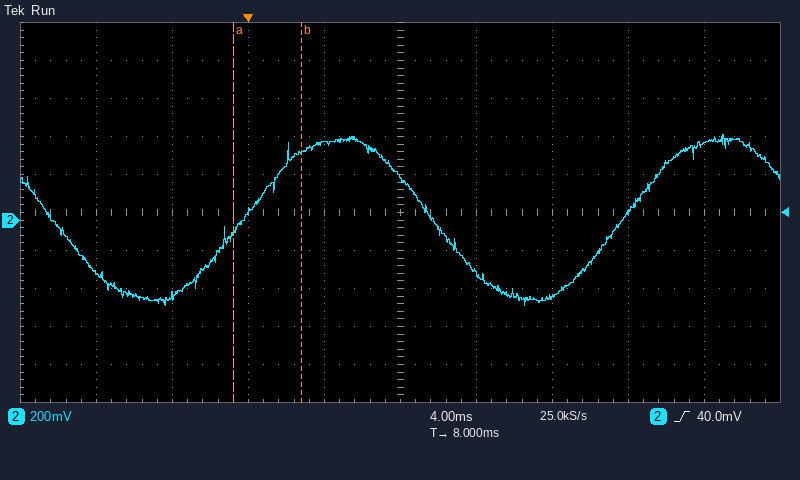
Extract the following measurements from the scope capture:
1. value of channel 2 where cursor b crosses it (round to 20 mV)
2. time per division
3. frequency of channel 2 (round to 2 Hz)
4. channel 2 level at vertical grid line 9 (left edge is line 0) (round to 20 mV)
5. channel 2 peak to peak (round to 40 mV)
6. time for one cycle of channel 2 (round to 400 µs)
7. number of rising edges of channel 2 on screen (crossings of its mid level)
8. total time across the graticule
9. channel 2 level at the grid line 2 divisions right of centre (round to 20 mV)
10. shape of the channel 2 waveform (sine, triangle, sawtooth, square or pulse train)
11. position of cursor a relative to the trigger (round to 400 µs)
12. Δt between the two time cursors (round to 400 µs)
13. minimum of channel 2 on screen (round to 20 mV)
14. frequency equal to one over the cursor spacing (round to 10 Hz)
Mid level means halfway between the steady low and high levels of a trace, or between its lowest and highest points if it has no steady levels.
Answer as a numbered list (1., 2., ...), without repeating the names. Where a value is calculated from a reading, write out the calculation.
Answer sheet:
1. 360 mV
2. 4 ms
3. 1 / 20.0 ms ≈ 50 Hz
4. 400 mV
5. 880 mV
6. 20.0 ms
7. 2
8. 40 ms
9. -400 mV
10. sine
11. -800 µs
12. 3.6 ms
13. -440 mV
14. 1 / 3.6 ms ≈ 280 Hz
